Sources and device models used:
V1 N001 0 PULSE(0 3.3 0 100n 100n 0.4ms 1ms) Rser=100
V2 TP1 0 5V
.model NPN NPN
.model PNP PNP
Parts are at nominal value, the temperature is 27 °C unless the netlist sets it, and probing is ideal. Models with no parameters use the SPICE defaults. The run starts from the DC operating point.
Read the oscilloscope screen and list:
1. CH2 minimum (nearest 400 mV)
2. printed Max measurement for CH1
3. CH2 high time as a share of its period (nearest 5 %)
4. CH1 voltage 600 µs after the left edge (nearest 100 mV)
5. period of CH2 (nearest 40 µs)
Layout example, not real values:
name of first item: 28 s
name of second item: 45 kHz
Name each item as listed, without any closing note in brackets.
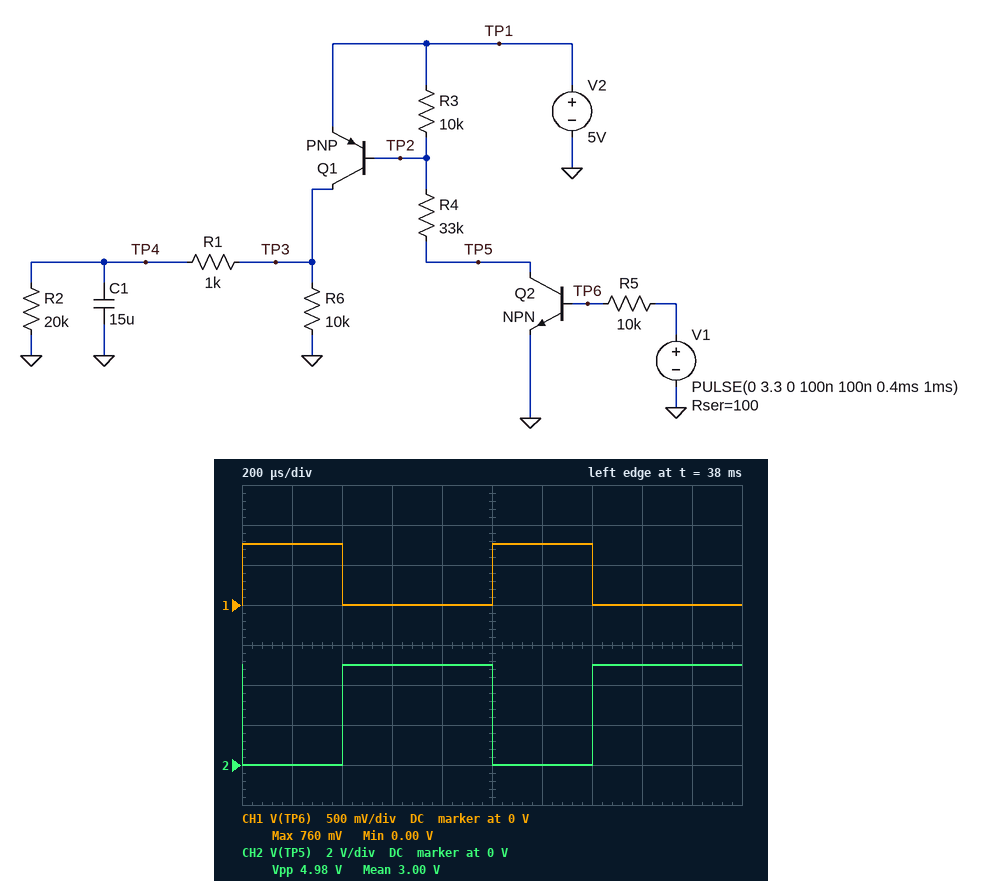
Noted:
CH2 minimum: 0 V
printed Max measurement for CH1: 760 mV
CH2 high time as a share of its period: 60 %
CH1 voltage 600 µs after the left edge: 0 V
period of CH2: 1.00 ms
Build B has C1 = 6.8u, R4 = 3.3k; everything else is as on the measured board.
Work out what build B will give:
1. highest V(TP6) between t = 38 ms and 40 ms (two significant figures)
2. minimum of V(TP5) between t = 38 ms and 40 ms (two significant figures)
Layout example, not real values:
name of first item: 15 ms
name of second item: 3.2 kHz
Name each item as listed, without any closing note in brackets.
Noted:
highest V(TP6) between t = 38 ms and 40 ms: 790 mV
minimum of V(TP5) between t = 38 ms and 40 ms: 52 mV
